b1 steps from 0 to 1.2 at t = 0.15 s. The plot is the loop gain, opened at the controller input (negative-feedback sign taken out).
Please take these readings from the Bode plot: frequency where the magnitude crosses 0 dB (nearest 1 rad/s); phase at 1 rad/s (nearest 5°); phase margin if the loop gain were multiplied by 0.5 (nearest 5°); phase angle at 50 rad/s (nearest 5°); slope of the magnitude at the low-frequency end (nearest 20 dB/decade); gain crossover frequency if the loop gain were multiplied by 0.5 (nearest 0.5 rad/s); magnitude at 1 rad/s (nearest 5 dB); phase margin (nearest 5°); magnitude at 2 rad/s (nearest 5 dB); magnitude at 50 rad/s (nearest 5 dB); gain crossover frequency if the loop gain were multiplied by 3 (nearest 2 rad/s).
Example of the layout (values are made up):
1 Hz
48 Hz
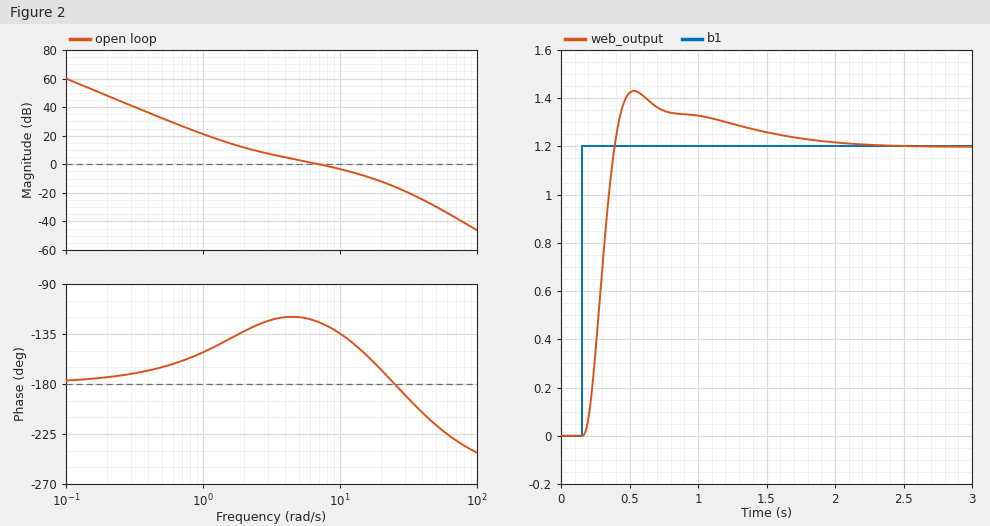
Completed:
7 rad/s
-150°
60°
-215°
-40 dB/decade
3.5 rad/s
20 dB
55°
10 dB
-30 dB
16 rad/s
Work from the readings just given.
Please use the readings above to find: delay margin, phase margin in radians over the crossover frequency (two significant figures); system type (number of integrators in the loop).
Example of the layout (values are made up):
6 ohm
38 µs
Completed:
0.14 s
2
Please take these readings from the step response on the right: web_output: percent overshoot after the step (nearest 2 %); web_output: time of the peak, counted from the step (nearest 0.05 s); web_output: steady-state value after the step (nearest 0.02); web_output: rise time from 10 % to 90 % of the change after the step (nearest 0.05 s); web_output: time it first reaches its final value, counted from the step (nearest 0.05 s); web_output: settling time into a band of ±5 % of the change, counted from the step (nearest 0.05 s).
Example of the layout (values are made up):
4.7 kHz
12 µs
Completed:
20 %
0.40 s
1.20
0.15 s
0.25 s
1.35 s
